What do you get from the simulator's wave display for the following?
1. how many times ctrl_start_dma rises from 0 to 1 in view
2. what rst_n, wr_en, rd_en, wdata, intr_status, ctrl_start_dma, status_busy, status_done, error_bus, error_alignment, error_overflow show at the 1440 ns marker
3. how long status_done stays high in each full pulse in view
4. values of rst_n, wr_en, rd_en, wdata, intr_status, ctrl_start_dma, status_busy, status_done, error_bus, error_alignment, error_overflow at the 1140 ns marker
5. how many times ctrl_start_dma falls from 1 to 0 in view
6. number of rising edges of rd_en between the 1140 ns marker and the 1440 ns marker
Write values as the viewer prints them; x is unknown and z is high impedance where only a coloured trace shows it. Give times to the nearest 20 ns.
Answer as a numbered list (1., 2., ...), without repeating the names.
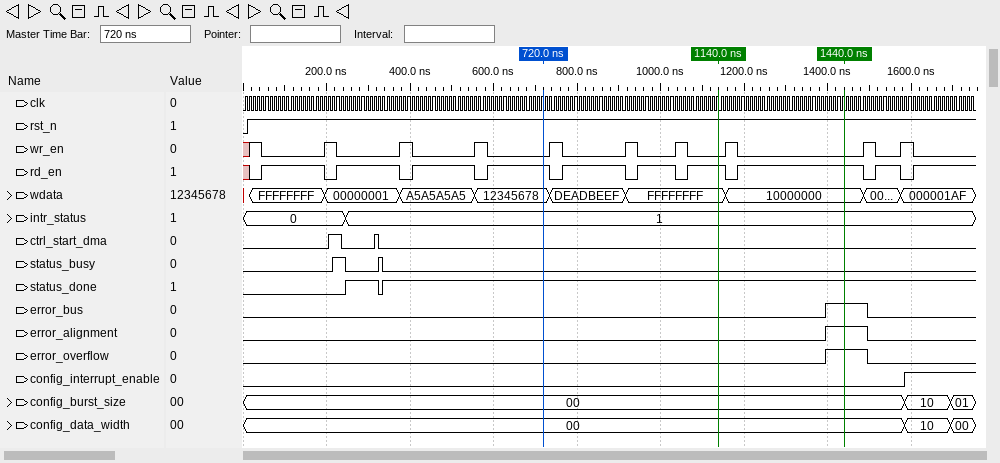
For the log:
1. 2
2. rst_n=1, wr_en=0, rd_en=1, wdata=10000000, intr_status=1, ctrl_start_dma=0, status_busy=0, status_done=1, error_bus=1, error_alignment=1, error_overflow=1
3. 80 ns
4. rst_n=1, wr_en=0, rd_en=1, wdata=FFFFFFFF, intr_status=1, ctrl_start_dma=0, status_busy=0, status_done=1, error_bus=0, error_alignment=0, error_overflow=0
5. 2
6. 1
